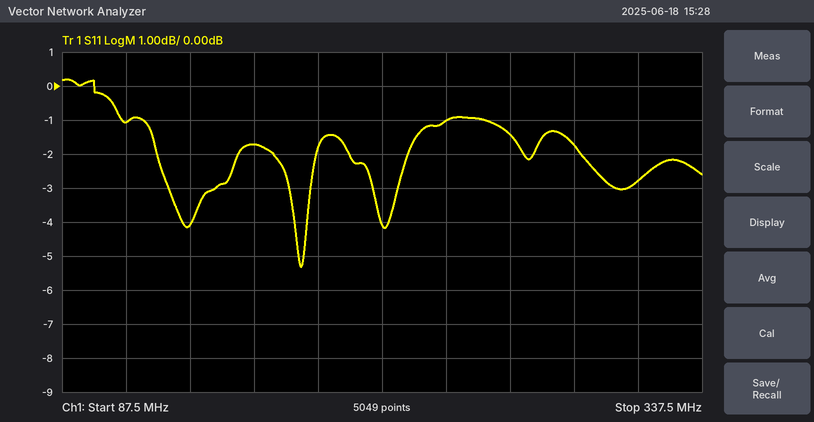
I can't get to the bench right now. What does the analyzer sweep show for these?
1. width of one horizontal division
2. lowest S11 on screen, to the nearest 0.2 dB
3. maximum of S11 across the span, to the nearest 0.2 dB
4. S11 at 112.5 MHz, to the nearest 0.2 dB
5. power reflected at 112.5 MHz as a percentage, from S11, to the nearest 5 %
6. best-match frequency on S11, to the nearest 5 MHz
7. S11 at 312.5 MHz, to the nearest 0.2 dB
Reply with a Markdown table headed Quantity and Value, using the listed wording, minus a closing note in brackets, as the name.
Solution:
| Quantity | Value |
|---|---|
| width of one horizontal division | 25 MHz |
| lowest S11 on screen, to the nearest 0.2 dB | -5.4 dB |
| maximum of S11 across the span, to the nearest 0.2 dB | 0.2 dB |
| S11 at 112.5 MHz, to the nearest 0.2 dB | -1.0 dB |
| power reflected at 112.5 MHz as a percentage, from S11, to the nearest 5 % | 80 % |
| best-match frequency on S11, to the nearest 5 MHz | 180 MHz |
| S11 at 312.5 MHz, to the nearest 0.2 dB | -2.8 dB |
